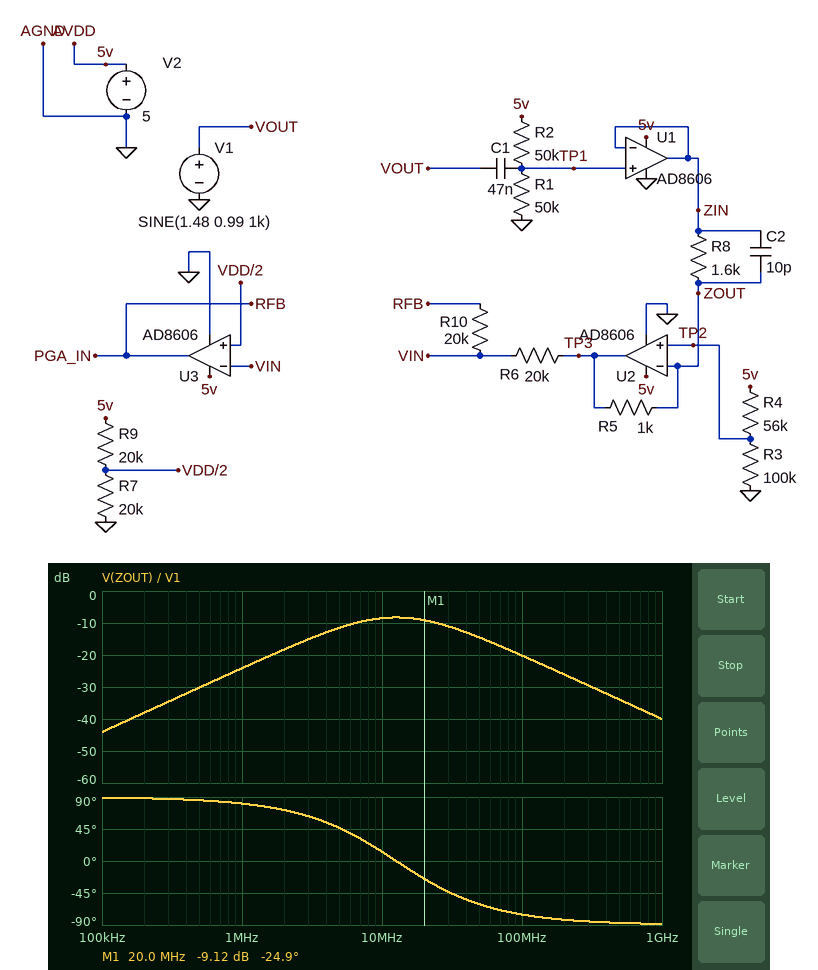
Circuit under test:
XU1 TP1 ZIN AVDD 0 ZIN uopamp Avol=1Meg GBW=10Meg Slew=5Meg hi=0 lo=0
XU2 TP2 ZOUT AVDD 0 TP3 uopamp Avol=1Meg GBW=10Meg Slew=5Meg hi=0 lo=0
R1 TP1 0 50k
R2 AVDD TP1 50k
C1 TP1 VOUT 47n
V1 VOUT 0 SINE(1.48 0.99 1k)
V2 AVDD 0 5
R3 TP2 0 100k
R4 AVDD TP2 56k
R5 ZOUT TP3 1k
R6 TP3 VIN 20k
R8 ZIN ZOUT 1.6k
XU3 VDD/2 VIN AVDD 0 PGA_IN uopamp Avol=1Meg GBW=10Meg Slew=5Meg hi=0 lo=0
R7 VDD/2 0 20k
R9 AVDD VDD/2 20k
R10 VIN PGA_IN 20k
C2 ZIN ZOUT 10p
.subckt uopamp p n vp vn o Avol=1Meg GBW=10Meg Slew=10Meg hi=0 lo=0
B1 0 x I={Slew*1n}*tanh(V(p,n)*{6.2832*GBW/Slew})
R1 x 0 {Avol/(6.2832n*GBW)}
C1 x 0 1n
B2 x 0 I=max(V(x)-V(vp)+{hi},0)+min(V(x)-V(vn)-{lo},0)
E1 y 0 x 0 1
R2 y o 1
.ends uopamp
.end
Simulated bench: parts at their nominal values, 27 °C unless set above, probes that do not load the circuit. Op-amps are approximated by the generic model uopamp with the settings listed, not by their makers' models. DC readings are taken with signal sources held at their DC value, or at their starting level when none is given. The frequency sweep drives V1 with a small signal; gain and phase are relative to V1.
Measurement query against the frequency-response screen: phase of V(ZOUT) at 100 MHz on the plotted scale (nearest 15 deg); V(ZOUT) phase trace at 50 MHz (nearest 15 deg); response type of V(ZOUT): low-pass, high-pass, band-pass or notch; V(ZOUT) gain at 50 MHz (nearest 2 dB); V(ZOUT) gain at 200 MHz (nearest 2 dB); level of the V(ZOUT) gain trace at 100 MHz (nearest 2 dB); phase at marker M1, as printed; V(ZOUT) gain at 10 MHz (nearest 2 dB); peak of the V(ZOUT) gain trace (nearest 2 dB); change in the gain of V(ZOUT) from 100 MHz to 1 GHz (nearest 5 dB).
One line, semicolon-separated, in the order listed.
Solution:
-75 deg; -60 deg; band-pass; -14 dB; -26 dB; -20 dB; -24.9 deg; -8 dB; -8 dB; -20 dB
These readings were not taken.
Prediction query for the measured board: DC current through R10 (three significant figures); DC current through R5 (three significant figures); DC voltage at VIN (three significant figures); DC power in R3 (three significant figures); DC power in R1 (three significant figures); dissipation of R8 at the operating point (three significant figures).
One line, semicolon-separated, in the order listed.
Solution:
57.3 µA; 441 µA; 2.50 V; 103 µW; 125 µW; 311 µW
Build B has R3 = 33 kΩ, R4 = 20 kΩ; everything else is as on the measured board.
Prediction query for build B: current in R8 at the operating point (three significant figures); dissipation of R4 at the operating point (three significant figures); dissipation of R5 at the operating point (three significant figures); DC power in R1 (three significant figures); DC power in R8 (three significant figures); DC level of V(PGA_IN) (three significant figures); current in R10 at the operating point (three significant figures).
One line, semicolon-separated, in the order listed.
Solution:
383 µA; 178 µW; 147 µW; 125 µW; 235 µW; 1.50 V; 49.8 µA
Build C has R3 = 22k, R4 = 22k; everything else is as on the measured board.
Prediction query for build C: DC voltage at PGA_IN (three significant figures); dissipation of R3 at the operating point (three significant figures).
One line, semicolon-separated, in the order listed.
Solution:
2.50 V; 284 µW
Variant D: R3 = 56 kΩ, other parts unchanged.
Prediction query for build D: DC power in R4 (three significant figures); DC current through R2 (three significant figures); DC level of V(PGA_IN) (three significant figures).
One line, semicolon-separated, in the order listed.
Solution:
112 µW; 50.0 µA; 2.50 V
